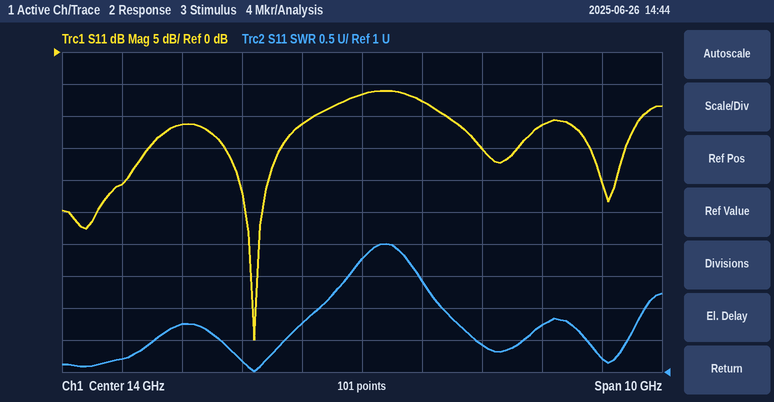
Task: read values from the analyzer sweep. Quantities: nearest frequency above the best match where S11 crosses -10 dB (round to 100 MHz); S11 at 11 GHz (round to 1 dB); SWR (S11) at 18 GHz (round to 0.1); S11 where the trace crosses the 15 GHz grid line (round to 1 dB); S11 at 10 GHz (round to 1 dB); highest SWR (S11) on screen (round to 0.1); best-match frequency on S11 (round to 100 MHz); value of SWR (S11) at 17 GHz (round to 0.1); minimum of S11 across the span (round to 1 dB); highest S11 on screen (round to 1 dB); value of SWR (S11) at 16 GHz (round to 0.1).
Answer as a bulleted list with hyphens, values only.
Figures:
- 13.2 GHz
- -11 dB
- 1.2
- -8 dB
- -21 dB
- 3.0
- 12.2 GHz
- 1.7
- -45 dB
- -6 dB
- 1.4
